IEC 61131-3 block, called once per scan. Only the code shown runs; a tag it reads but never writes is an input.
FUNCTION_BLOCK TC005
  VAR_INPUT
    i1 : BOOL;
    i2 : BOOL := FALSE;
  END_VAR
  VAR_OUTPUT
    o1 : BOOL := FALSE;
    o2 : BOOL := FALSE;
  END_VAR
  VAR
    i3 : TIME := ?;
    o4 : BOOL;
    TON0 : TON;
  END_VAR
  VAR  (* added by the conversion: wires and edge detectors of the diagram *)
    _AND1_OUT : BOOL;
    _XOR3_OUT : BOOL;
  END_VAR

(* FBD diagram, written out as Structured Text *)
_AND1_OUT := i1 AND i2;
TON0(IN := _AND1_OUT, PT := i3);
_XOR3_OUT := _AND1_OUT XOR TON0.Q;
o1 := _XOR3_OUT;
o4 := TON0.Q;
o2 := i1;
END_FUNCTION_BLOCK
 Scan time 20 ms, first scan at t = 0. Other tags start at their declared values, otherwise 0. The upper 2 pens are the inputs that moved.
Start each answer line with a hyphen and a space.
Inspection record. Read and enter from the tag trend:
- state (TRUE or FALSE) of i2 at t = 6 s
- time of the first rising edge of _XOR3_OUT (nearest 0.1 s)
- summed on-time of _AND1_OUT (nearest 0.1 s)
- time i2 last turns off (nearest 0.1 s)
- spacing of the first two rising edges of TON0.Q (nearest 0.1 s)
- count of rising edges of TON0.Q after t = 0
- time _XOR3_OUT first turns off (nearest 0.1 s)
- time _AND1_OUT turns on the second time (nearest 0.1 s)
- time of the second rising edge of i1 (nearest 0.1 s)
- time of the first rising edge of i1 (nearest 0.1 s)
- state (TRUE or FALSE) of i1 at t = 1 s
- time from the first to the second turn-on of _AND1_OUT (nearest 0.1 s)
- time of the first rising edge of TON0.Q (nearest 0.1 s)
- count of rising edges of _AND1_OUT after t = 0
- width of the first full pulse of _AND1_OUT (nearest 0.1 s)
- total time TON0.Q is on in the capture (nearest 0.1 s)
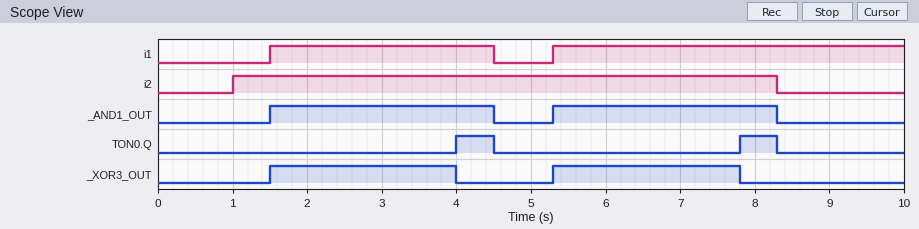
- TRUE
- 1.5 s
- 6.0 s
- 8.3 s
- 3.8 s
- 2
- 4.0 s
- 5.3 s
- 5.3 s
- 1.5 s
- FALSE
- 3.8 s
- 4.0 s
- 2
- 3.0 s
- 1.0 s
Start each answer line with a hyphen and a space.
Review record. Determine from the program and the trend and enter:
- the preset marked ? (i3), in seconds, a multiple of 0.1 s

- 2.5 s
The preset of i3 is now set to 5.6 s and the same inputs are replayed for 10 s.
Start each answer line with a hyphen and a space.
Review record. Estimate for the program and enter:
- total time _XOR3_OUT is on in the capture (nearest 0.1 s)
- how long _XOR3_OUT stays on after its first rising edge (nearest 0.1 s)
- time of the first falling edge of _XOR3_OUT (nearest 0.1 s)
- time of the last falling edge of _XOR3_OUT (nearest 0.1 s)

- 6.0 s
- 3.0 s
- 4.5 s
- 8.3 s
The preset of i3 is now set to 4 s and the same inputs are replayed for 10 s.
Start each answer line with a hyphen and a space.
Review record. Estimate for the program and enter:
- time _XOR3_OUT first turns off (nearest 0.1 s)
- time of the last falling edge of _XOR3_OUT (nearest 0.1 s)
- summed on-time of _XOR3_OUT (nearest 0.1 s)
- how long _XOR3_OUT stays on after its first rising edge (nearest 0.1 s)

- 4.5 s
- 8.3 s
- 6.0 s
- 3.0 s
